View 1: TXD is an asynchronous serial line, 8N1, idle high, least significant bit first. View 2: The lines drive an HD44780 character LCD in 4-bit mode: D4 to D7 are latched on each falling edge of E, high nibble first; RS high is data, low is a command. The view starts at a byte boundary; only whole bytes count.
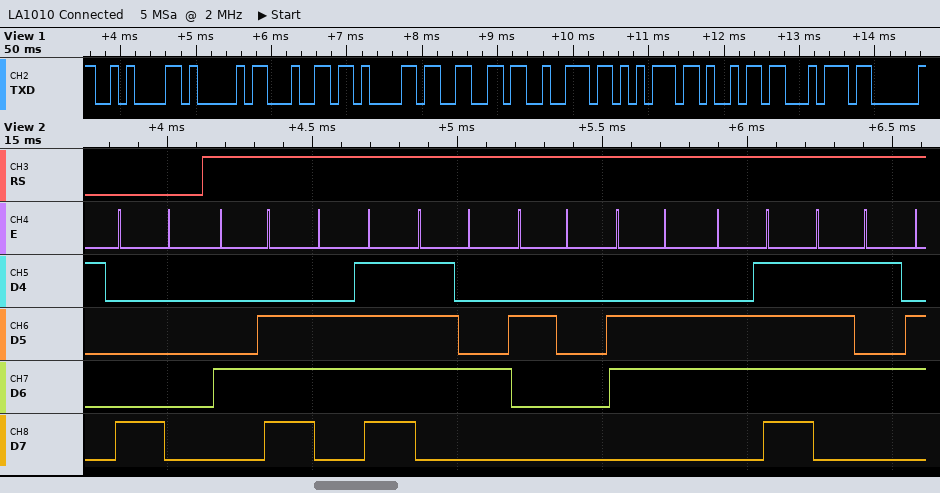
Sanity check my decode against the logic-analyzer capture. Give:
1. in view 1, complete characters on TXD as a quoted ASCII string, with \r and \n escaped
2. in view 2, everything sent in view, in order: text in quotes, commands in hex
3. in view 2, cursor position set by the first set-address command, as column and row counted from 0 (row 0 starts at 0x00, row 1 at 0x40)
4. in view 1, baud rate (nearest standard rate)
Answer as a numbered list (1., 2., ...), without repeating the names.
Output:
1. "\nAdafruit"
2. 0x80 "Not fou"
3. column 0, row 0
4. 9600 baud
